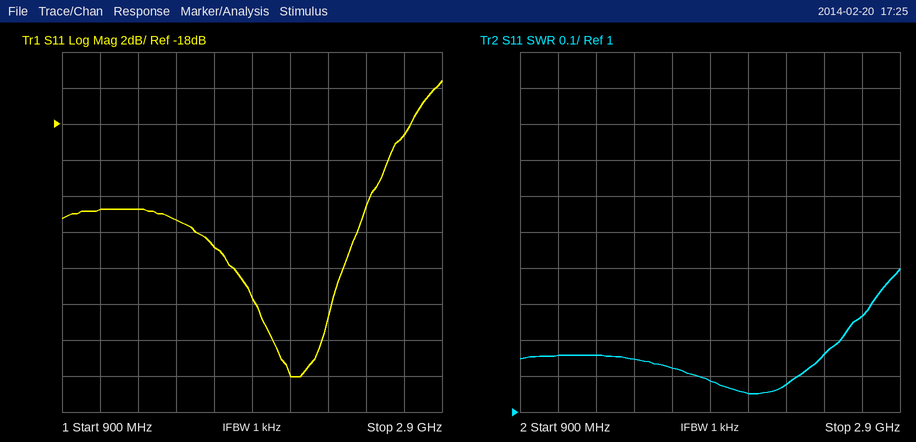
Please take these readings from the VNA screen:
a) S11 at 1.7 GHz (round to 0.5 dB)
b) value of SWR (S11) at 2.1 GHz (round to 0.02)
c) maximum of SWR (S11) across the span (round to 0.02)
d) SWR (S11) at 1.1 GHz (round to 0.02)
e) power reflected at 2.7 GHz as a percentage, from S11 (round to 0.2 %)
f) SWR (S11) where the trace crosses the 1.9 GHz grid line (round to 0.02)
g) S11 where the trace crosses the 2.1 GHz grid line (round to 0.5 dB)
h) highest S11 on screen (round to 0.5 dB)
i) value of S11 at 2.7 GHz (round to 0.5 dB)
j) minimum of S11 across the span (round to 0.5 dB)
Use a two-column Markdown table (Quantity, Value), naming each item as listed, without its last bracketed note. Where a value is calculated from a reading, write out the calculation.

| Quantity | Value |
|---|---|
| S11 at 1.7 GHz | -25.0 dB |
| value of SWR (S11) at 2.1 GHz | 1.06 |
| maximum of SWR (S11) across the span | 1.40 |
| SWR (S11) at 1.1 GHz | 1.16 |
| power reflected at 2.7 GHz as a percentage, from S11 | 10^(-18.5/10) ≈ 1.4 % |
| SWR (S11) where the trace crosses the 1.9 GHz grid line | 1.08 |
| S11 where the trace crosses the 2.1 GHz grid line | -32.0 dB |
| highest S11 on screen | -15.5 dB |
| value of S11 at 2.7 GHz | -18.5 dB |
| minimum of S11 across the span | -32.0 dB |
